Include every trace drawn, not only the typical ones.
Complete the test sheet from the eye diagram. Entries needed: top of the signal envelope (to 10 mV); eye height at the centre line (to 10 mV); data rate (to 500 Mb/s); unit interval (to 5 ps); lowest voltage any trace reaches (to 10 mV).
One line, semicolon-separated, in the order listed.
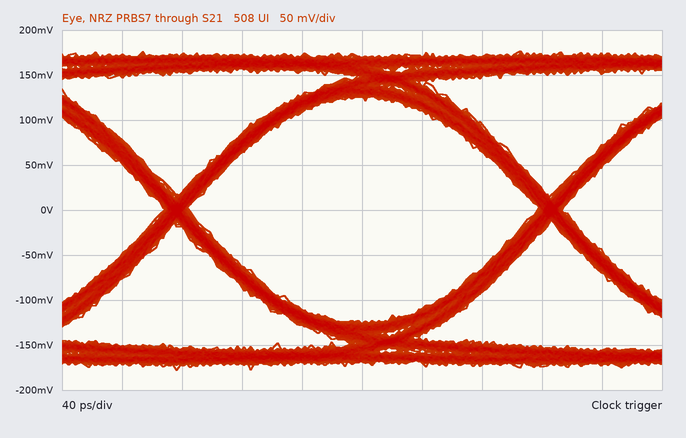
180 mV; 250 mV; 4.0 Gb/s; 250 ps; -180 mV
